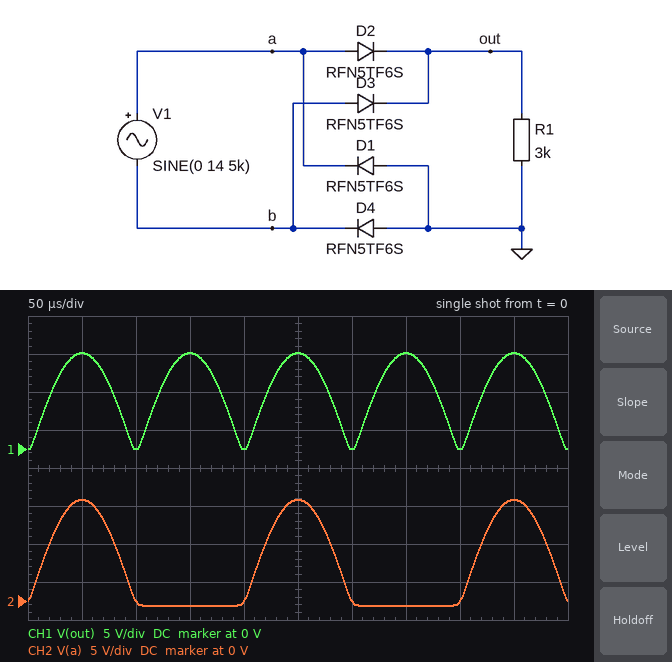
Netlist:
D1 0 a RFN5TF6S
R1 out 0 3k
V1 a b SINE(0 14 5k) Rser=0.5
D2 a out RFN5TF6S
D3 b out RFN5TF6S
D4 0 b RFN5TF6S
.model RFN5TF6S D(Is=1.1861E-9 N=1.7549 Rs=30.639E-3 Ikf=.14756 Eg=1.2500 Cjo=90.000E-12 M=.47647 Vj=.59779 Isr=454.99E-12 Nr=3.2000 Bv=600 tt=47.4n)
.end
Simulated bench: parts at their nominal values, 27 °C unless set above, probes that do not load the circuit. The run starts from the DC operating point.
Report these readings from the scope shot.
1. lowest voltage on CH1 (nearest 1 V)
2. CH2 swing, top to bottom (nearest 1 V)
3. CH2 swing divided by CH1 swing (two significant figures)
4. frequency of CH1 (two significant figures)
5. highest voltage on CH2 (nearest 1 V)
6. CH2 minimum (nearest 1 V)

0 V
14 V
1.1
10 kHz
13 V
-1 V
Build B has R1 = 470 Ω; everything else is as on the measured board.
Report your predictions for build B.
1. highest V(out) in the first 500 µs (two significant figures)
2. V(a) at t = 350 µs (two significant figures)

12 V
-790 mV
